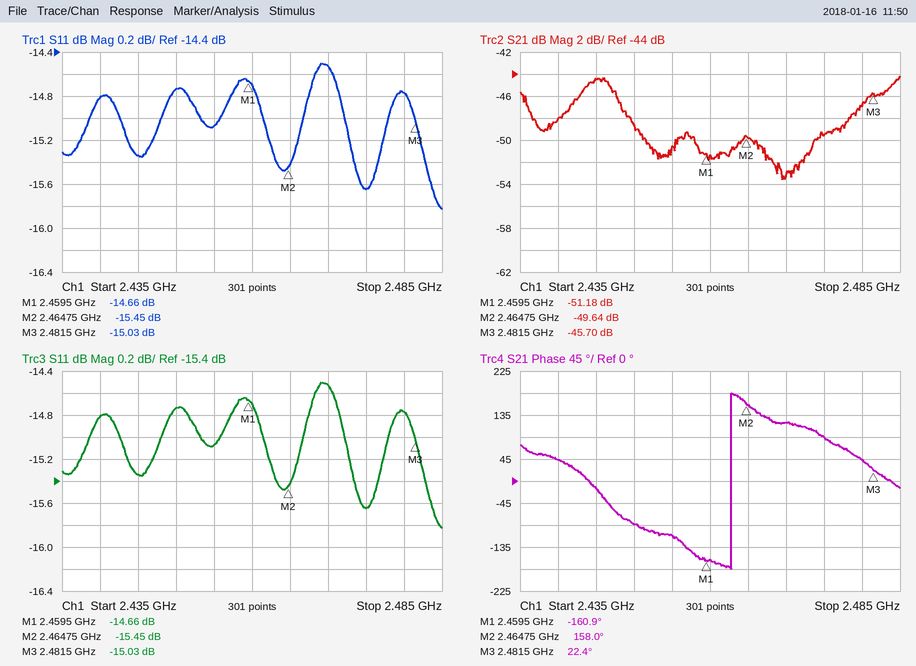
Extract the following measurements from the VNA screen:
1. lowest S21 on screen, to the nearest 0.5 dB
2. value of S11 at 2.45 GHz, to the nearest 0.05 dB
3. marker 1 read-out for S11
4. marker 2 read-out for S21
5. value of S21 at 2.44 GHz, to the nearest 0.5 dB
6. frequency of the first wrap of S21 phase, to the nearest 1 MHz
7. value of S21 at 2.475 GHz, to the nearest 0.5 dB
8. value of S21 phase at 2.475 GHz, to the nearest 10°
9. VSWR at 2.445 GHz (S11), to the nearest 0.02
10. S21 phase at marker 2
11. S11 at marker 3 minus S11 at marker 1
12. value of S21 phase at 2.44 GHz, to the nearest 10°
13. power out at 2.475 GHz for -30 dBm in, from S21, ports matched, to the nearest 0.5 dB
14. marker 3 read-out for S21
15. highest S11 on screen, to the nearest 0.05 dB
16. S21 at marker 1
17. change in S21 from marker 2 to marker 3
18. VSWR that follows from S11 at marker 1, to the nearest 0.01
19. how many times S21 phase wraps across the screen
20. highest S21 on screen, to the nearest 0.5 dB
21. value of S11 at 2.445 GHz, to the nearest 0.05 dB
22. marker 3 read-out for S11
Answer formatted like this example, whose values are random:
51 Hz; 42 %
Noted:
-53.5 dB; -14.75 dB; -14.66 dB; -49.64 dB; -48.0 dB; 2.463 GHz; -49.5 dB; 90°; 1.42; 158.0°; -0.37 dB; 40°; -79.5 dBm; -45.70 dB; -14.50 dB; -51.18 dB; 3.94 dB; 1.45; 1; -44.0 dB; -15.35 dB; -15.03 dB
